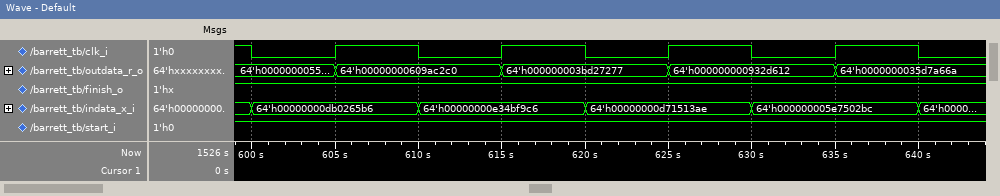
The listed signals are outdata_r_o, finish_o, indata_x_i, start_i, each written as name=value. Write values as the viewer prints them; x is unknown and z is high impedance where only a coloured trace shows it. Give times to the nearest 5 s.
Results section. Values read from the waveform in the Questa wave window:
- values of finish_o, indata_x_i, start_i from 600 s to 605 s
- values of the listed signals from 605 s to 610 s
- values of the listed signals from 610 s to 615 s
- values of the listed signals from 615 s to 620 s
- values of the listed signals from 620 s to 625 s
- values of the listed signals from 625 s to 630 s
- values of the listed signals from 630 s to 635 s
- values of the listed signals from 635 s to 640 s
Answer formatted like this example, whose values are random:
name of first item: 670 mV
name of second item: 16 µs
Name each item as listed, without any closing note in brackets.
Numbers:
values of finish_o, indata_x_i, start_i from 600 s to 605 s: finish_o=1, indata_x_i=64'h00000000db0265b6, start_i=1
values of the listed signals from 605 s to 610 s: outdata_r_o=64'h00000000609ac2c0, finish_o=1, indata_x_i=64'h00000000db0265b6, start_i=1
values of the listed signals from 610 s to 615 s: outdata_r_o=64'h00000000609ac2c0, finish_o=1, indata_x_i=64'h00000000e34bf9c6, start_i=1
values of the listed signals from 615 s to 620 s: outdata_r_o=64'h000000003bd27277, finish_o=1, indata_x_i=64'h00000000e34bf9c6, start_i=1
values of the listed signals from 620 s to 625 s: outdata_r_o=64'h000000003bd27277, finish_o=1, indata_x_i=64'h00000000d71513ae, start_i=1
values of the listed signals from 625 s to 630 s: outdata_r_o=64'h000000000932d612, finish_o=1, indata_x_i=64'h00000000d71513ae, start_i=1
values of the listed signals from 630 s to 635 s: outdata_r_o=64'h000000000932d612, finish_o=1, indata_x_i=64'h000000005e7502bc, start_i=1
values of the listed signals from 635 s to 640 s: outdata_r_o=64'h0000000035d7a66a, finish_o=1, indata_x_i=64'h000000005e7502bc, start_i=1
